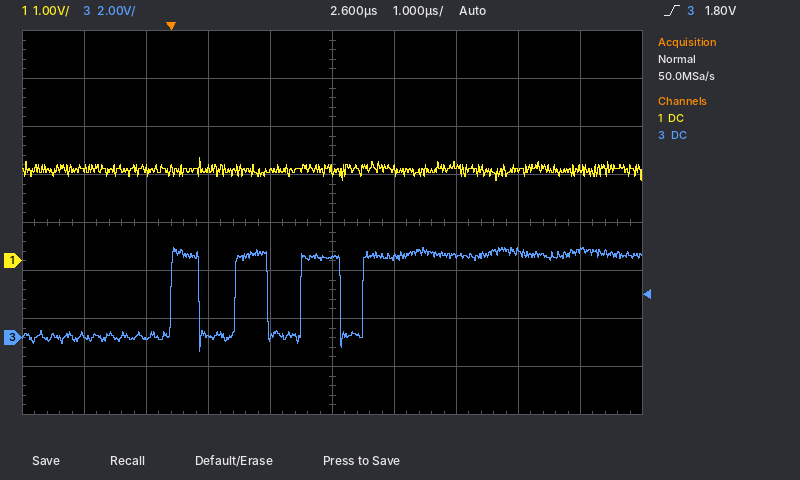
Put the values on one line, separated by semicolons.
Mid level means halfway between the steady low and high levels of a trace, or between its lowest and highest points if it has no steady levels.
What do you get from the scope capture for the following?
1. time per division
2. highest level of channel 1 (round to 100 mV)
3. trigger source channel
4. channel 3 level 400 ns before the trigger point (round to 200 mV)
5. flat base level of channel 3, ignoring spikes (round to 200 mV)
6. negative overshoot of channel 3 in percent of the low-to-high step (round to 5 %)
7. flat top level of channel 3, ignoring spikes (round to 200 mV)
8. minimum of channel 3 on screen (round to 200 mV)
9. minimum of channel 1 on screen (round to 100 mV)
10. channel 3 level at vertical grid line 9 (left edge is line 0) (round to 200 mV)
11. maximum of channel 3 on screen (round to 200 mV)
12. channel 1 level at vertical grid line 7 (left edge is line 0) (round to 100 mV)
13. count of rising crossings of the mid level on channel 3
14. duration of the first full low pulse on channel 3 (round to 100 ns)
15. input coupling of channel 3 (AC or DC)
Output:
1 µs; 2.2 V; channel 3; 0.0 V; 0.0 V; 20 %; 3.4 V; -600 mV; 1.7 V; 3.6 V; 3.8 V; 2.0 V; 4; 600 ns; DC
